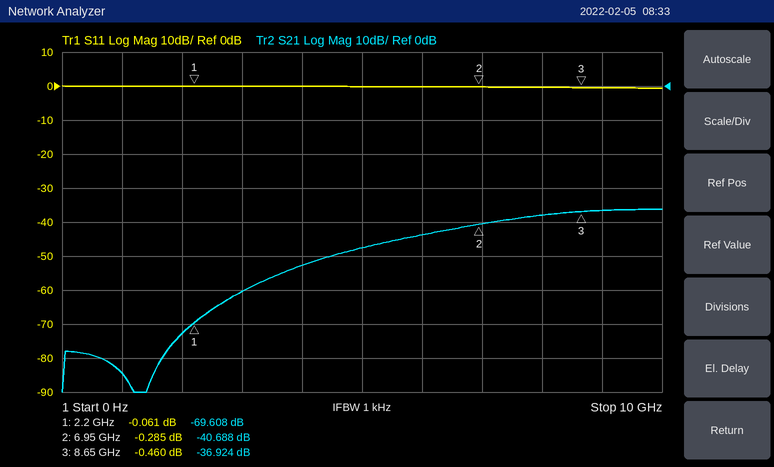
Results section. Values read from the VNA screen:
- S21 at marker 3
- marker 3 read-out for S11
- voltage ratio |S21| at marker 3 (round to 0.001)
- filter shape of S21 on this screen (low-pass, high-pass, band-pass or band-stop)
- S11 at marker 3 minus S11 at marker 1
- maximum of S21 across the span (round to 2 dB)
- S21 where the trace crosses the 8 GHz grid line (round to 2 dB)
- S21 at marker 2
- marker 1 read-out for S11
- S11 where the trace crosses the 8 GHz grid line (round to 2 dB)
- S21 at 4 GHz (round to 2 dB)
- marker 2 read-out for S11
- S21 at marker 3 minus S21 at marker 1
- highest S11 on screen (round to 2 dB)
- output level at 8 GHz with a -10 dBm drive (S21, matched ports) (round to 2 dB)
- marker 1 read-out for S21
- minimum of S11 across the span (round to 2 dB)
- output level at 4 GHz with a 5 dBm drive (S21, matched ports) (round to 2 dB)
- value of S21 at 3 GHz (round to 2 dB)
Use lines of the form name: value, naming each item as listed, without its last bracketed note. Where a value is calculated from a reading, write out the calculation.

S21 at marker 3: -36.924 dB
marker 3 read-out for S11: -0.460 dB
voltage ratio |S21| at marker 3: 10^(-36.924/20) ≈ 0.014
filter shape of S21 on this screen: high-pass
S11 at marker 3 minus S11 at marker 1: -0.46 − (-0.061) = -0.399 dB
maximum of S21 across the span: -36 dB
S21 where the trace crosses the 8 GHz grid line: -38 dB
S21 at marker 2: -40.688 dB
marker 1 read-out for S11: -0.061 dB
S11 where the trace crosses the 8 GHz grid line: 0 dB
S21 at 4 GHz: -52 dB
marker 2 read-out for S11: -0.285 dB
S21 at marker 3 minus S21 at marker 1: -36.924 − (-69.608) = 32.684 dB
highest S11 on screen: 0 dB
output level at 8 GHz with a -10 dBm drive (S21, matched ports): -10 dBm + (-38 dB) = -48 dBm
marker 1 read-out for S21: -69.608 dB
minimum of S11 across the span: 0 dB
output level at 4 GHz with a 5 dBm drive (S21, matched ports): 5 dBm + (-52 dB) = -48 dBm
value of S21 at 3 GHz: -60 dB
